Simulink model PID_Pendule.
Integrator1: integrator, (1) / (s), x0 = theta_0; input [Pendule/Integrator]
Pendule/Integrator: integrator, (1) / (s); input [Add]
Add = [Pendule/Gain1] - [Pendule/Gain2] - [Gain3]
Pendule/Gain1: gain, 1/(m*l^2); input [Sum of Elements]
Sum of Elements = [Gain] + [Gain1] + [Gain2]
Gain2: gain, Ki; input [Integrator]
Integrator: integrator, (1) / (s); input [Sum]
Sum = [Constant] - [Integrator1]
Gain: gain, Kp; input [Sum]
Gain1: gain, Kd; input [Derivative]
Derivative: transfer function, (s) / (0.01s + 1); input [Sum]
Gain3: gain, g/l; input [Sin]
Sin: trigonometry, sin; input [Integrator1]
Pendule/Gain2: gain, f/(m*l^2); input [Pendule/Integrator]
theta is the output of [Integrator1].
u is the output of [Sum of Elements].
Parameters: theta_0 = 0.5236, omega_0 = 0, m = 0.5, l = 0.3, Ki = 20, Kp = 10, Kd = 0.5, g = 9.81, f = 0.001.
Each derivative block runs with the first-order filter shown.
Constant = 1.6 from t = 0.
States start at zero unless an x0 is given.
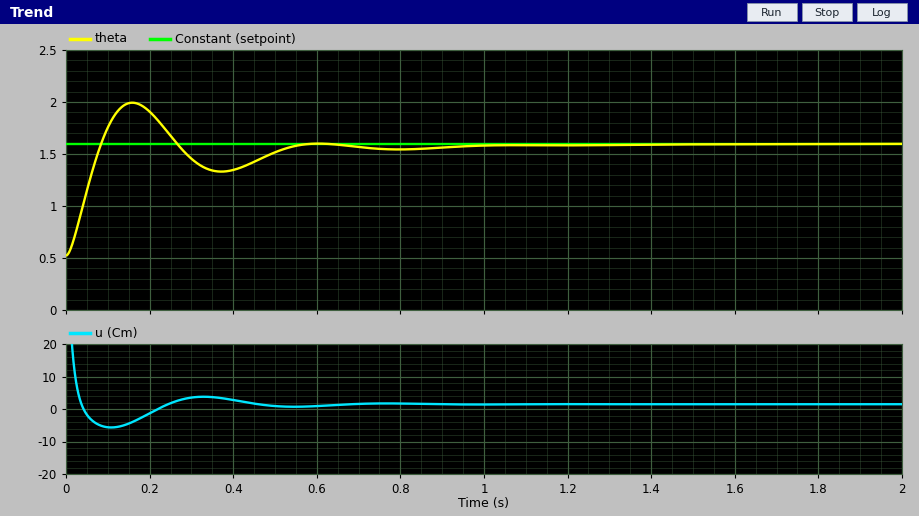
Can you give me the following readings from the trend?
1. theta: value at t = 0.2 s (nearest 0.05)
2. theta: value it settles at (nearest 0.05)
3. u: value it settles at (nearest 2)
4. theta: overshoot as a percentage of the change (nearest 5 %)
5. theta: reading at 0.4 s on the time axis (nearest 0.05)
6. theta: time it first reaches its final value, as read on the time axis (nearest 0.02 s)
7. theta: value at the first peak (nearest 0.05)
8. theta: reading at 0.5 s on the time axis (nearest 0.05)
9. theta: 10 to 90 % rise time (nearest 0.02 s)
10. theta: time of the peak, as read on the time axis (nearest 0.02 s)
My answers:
1.90
1.60
2
35 %
1.35
0.08 s
2.00
1.50
0.06 s
0.16 s
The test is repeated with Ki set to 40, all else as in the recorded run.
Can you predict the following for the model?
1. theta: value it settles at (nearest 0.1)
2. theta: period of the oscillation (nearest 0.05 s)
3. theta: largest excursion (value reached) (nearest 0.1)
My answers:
1.6
0.45 s
2.1
